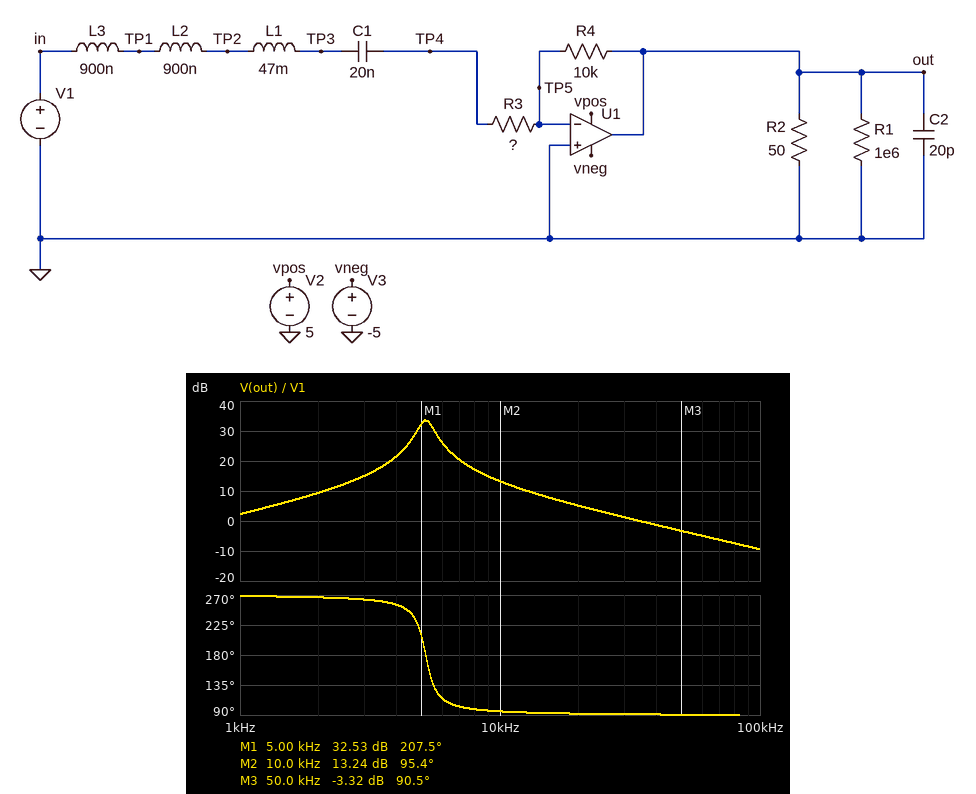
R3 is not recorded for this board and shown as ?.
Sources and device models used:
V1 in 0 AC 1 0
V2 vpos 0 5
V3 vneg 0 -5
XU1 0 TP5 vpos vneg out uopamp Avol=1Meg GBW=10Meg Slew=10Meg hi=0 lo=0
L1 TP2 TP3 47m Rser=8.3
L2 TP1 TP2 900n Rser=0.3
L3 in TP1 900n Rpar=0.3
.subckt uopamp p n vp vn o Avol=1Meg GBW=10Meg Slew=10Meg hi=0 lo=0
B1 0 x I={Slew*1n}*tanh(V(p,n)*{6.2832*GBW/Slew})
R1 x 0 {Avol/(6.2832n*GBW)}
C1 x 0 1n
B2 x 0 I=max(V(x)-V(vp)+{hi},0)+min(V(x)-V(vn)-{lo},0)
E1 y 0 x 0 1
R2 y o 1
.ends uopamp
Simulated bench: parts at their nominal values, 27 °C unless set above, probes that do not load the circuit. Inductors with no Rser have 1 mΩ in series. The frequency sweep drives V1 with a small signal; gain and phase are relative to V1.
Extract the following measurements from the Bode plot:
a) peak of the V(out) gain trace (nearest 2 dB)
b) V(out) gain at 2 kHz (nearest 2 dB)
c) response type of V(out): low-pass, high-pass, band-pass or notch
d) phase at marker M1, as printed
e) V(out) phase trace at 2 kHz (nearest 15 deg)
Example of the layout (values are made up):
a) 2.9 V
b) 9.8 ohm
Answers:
a) 34 dB
b) 10 dB
c) band-pass
d) 207.5 deg
e) 270 deg
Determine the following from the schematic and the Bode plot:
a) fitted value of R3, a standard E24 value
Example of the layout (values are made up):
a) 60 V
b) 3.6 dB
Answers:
a) 200 Ω
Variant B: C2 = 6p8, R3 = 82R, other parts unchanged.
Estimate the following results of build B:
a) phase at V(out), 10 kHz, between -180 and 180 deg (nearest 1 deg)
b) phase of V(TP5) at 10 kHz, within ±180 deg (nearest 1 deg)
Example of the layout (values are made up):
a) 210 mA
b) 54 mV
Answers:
a) 92 deg
b) 2 deg
